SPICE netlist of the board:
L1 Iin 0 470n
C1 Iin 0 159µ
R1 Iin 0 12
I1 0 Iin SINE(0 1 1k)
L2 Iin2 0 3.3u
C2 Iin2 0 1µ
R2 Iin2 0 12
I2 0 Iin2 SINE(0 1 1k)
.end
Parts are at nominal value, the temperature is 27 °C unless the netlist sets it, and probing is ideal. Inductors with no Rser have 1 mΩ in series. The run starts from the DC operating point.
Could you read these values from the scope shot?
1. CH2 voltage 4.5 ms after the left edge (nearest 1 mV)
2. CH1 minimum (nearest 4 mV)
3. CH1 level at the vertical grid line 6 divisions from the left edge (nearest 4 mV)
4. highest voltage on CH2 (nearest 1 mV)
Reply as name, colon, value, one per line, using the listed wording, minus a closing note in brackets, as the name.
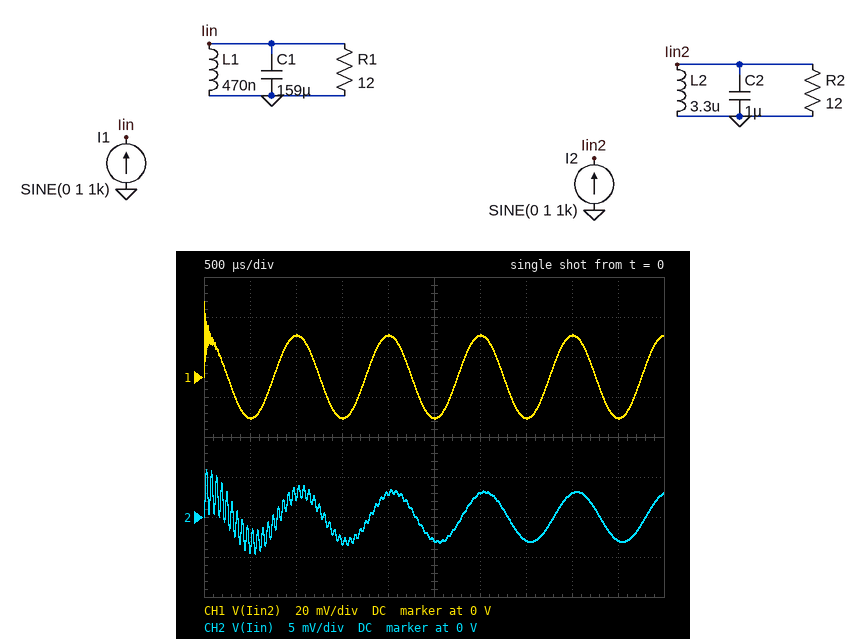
CH2 voltage 4.5 ms after the left edge: -3 mV
CH1 minimum: -20 mV
CH1 level at the vertical grid line 6 divisions from the left edge: 20 mV
highest voltage on CH2: 6 mV
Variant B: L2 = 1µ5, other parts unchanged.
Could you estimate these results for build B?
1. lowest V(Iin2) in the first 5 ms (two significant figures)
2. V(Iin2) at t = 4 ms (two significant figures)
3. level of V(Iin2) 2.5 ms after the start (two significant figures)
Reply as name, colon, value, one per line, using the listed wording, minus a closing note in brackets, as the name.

lowest V(Iin2) in the first 5 ms: -9.5 mV
V(Iin2) at t = 4 ms: 9.4 mV
level of V(Iin2) 2.5 ms after the start: -9.4 mV
